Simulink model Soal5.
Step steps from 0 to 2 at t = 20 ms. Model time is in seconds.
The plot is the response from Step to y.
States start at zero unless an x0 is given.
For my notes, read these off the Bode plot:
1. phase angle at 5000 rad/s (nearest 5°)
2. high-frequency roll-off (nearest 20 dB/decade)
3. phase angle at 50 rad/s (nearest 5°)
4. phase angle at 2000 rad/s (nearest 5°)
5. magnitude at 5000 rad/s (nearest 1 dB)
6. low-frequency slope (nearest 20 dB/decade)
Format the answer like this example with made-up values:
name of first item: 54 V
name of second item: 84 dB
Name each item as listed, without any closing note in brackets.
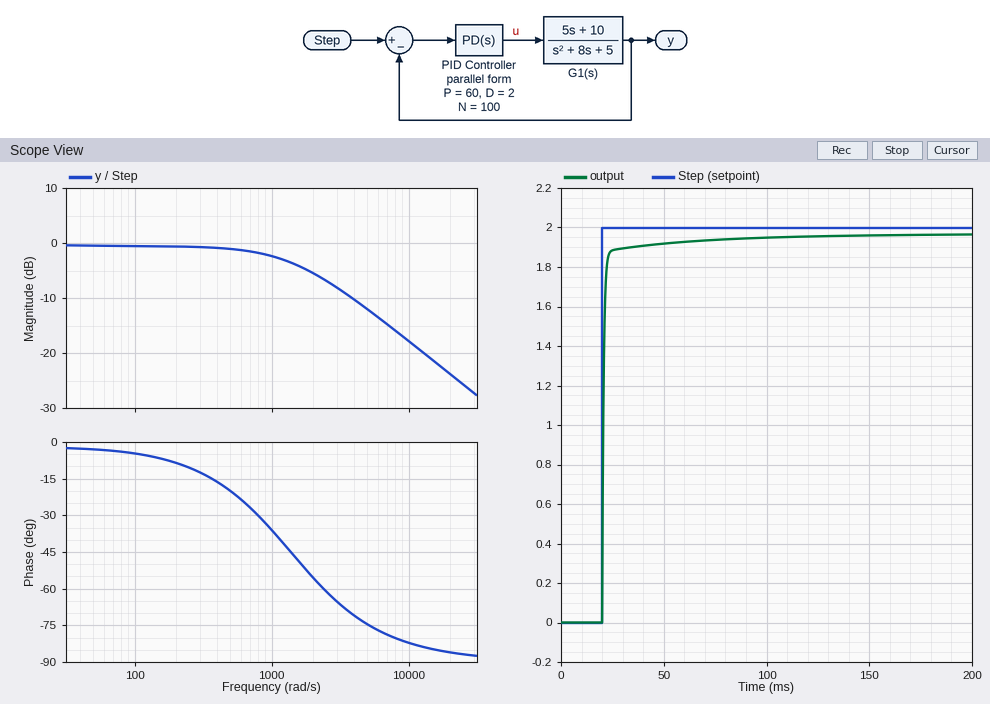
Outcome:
phase angle at 5000 rad/s: -75°
high-frequency roll-off: -20 dB/decade
phase angle at 50 rad/s: -5°
phase angle at 2000 rad/s: -55°
magnitude at 5000 rad/s: -12 dB
low-frequency slope: 0 dB/decade
